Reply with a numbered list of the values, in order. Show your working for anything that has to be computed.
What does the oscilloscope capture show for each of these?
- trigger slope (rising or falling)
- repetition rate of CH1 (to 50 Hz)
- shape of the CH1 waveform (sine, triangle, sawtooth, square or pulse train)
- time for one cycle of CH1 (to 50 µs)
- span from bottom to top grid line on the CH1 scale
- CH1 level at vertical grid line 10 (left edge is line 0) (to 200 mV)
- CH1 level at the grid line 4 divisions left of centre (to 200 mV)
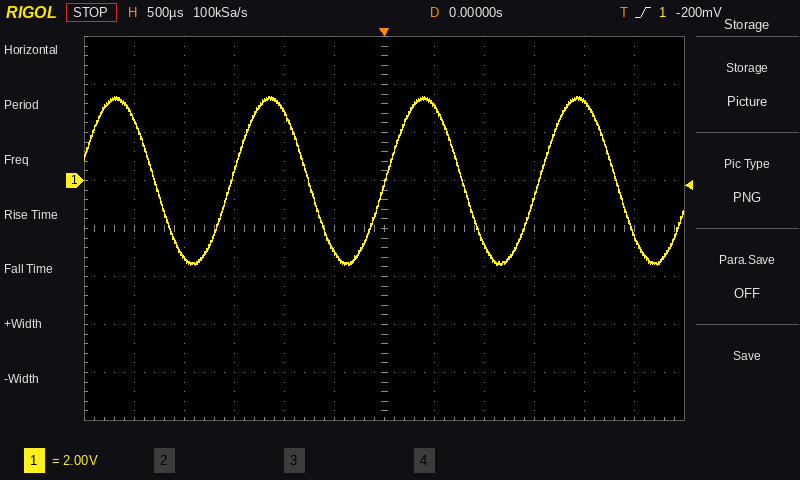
1. rising
2. 1 / 1.55 ms ≈ 645 Hz, so 650 Hz to the nearest 50 Hz
3. sine
4. 1.55 ms
5. 16 V
6. 3.2 V
7. -3.2 V
